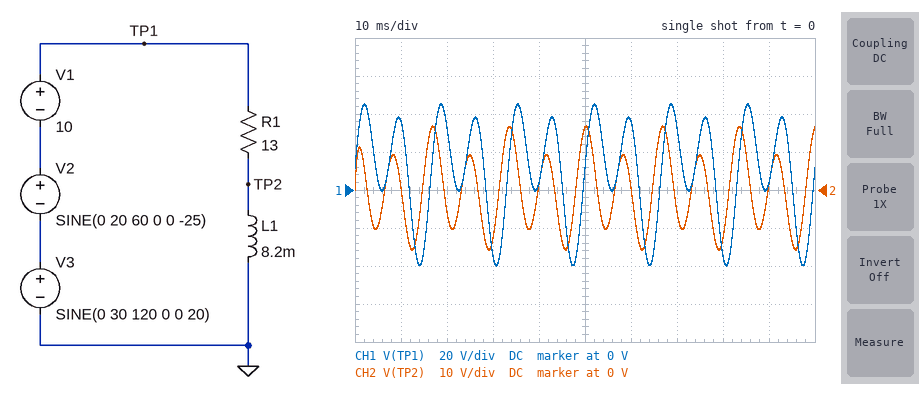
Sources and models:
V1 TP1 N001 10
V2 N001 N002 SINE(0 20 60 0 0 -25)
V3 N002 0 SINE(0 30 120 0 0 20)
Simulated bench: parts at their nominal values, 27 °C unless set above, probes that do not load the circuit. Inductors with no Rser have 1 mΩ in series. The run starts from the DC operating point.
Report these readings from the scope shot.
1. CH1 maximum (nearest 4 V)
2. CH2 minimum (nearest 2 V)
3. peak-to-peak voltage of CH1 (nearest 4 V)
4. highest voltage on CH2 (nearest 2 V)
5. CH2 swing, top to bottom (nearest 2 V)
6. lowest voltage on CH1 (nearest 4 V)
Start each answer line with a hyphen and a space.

- 44 V
- -16 V
- 84 V
- 16 V
- 32 V
- -40 V
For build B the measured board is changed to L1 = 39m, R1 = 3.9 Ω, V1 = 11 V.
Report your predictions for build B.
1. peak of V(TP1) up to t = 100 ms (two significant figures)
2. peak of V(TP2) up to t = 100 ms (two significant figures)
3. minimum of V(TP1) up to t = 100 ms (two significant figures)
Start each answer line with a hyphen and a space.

- 46 V
- 38 V
- -39 V
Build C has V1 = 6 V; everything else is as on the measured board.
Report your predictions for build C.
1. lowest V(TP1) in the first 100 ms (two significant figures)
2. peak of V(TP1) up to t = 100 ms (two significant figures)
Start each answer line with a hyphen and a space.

- -44 V
- 41 V
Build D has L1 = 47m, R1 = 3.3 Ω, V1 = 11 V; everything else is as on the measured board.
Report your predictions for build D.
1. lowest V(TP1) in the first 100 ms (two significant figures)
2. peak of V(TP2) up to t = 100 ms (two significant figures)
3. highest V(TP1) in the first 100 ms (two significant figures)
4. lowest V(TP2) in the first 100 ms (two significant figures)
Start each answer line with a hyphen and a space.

- -39 V
- 37 V
- 46 V
- -52 V
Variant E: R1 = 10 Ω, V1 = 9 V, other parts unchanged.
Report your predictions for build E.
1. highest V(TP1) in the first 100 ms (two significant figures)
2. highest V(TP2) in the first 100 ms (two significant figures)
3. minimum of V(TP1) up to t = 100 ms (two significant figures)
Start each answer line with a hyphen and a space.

- 44 V
- 21 V
- -41 V
